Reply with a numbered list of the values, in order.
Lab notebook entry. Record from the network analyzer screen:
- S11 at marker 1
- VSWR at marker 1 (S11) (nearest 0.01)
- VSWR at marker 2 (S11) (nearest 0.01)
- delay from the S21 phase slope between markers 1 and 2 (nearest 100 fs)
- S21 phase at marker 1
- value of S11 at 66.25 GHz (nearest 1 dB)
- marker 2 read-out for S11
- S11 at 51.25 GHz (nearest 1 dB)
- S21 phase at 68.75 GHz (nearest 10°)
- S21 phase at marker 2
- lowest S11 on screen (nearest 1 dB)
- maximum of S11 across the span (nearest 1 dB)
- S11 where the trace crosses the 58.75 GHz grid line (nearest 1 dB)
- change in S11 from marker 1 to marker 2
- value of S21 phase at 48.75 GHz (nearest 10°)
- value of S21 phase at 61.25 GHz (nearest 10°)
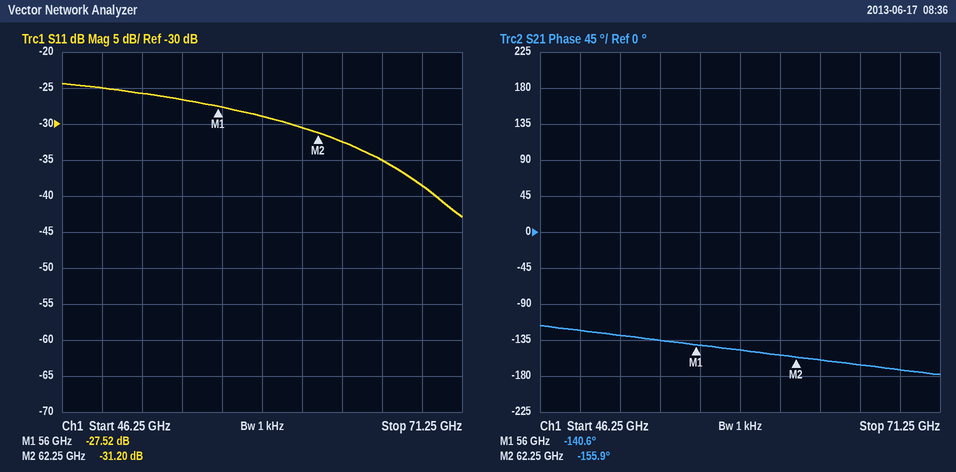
1. -27.52 dB
2. 1.09
3. 1.06
4. 6.8 ps
5. -140.6°
6. -35 dB
7. -31.20 dB
8. -26 dB
9. -170°
10. -155.9°
11. -43 dB
12. -24 dB
13. -29 dB
14. -3.68 dB
15. -120°
16. -150°
